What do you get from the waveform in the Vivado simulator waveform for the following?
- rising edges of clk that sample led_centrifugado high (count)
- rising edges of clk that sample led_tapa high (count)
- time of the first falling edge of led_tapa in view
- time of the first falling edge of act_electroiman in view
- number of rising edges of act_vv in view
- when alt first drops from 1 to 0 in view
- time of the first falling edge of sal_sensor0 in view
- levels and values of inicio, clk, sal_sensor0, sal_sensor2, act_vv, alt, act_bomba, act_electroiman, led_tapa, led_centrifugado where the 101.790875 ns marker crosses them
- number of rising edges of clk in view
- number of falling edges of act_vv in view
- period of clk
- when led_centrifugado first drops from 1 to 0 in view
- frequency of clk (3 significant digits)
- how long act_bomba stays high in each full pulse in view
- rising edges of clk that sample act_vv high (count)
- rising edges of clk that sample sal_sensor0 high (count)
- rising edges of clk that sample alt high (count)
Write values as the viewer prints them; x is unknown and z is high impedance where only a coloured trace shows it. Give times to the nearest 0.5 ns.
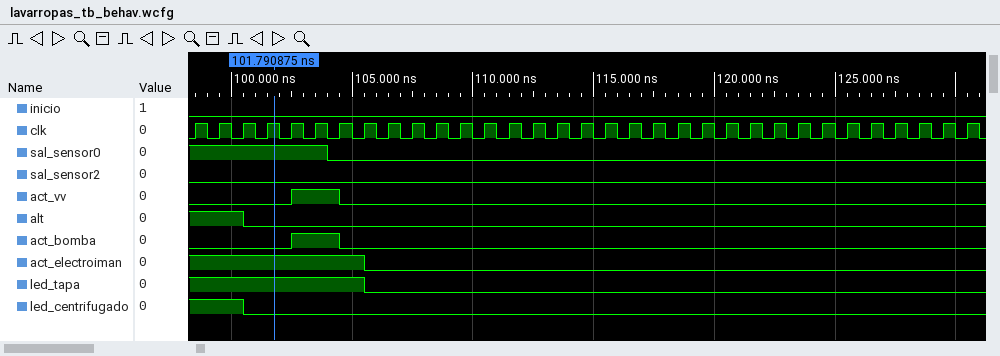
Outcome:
3
8
105.5 ns
105.5 ns
1
100.5 ns
104 ns
inicio=0, clk=1, sal_sensor0=1, sal_sensor2=0, act_vv=0, alt=0, act_bomba=0, act_electroiman=1, led_tapa=1, led_centrifugado=0
33
1
1 ns
100.5 ns
1.00 GHz
2 ns
2
6
3
